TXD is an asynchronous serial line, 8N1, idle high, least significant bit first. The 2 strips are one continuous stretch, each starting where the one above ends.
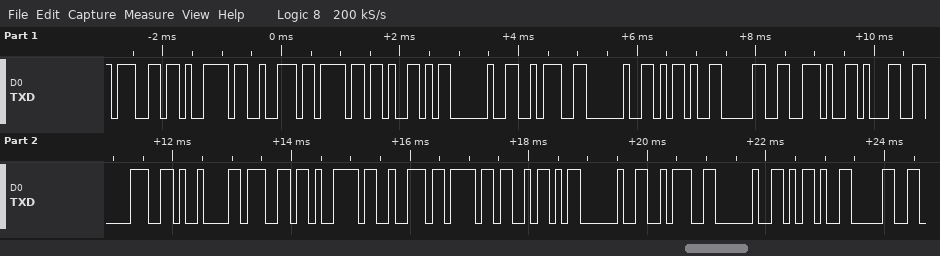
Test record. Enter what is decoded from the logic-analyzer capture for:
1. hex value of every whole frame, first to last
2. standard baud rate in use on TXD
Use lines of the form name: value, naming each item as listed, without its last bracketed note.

hex value of every whole frame, first to last: 67 79 72 6F 59 20 3A 20 2D 30 2E 31 38 09 67 79 72 6F 5A 20 3A 20 2D 30
standard baud rate in use on TXD: 9600 baud
